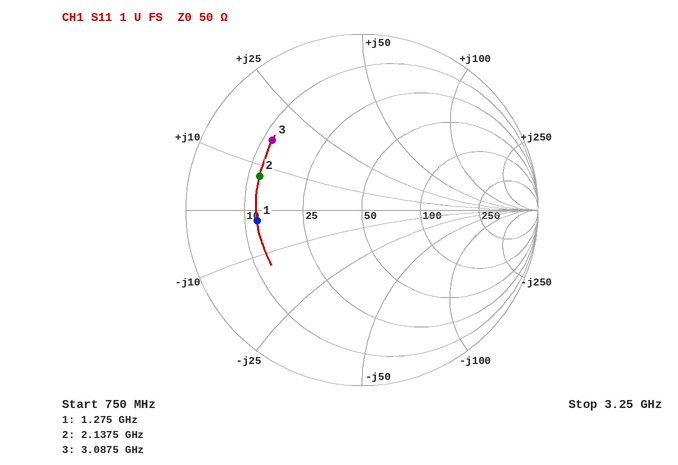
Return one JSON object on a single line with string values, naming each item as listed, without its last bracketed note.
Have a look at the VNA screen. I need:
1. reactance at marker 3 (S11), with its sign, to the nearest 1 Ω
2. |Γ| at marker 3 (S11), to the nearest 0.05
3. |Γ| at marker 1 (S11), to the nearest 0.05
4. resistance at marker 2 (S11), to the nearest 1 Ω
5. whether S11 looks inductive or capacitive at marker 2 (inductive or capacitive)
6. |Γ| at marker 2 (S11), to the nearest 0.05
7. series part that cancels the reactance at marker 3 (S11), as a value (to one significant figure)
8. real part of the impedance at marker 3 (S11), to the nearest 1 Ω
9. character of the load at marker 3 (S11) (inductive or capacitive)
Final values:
{"reactance at marker 3 (S11), with its sign, to the nearest 1 Ω": "+16 Ω", "|Γ| at marker 3 (S11), to the nearest 0.05": "0.65", "|Γ| at marker 1 (S11), to the nearest 0.05": "0.60", "resistance at marker 2 (S11), to the nearest 1 Ω": "12 Ω", "whether S11 looks inductive or capacitive at marker 2": "inductive", "|Γ| at marker 2 (S11), to the nearest 0.05": "0.60", "series part that cancels the reactance at marker 3 (S11), as a value": "3 pF", "real part of the impedance at marker 3 (S11), to the nearest 1 Ω": "12 Ω", "character of the load at marker 3 (S11)": "inductive"}
